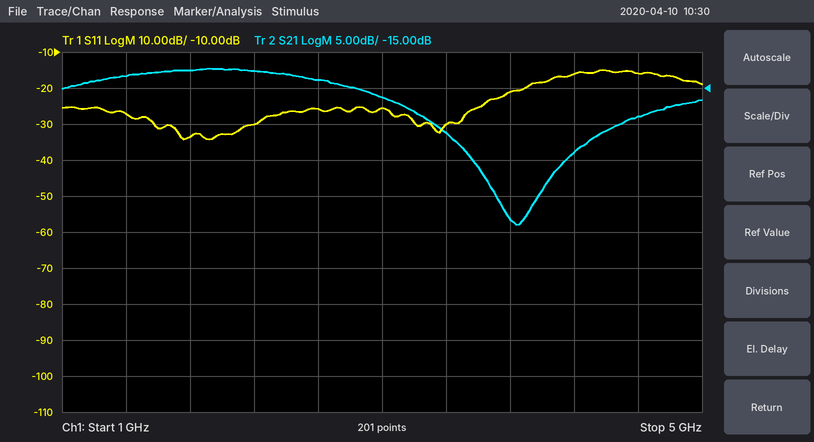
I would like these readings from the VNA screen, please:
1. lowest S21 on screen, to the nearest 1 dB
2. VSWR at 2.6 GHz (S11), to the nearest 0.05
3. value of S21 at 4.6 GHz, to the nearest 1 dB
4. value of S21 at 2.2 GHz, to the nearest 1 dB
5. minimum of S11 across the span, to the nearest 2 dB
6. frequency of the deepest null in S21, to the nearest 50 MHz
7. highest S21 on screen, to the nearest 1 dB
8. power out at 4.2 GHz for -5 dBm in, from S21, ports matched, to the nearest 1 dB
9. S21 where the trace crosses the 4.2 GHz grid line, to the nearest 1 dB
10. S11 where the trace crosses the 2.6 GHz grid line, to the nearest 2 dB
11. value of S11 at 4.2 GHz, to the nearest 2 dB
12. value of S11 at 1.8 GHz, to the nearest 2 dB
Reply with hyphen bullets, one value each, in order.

- -34 dB
- 1.10
- -19 dB
- -13 dB
- -34 dB
- 3.85 GHz
- -12 dB
- -29 dBm
- -24 dB
- -26 dB
- -16 dB
- -34 dB
